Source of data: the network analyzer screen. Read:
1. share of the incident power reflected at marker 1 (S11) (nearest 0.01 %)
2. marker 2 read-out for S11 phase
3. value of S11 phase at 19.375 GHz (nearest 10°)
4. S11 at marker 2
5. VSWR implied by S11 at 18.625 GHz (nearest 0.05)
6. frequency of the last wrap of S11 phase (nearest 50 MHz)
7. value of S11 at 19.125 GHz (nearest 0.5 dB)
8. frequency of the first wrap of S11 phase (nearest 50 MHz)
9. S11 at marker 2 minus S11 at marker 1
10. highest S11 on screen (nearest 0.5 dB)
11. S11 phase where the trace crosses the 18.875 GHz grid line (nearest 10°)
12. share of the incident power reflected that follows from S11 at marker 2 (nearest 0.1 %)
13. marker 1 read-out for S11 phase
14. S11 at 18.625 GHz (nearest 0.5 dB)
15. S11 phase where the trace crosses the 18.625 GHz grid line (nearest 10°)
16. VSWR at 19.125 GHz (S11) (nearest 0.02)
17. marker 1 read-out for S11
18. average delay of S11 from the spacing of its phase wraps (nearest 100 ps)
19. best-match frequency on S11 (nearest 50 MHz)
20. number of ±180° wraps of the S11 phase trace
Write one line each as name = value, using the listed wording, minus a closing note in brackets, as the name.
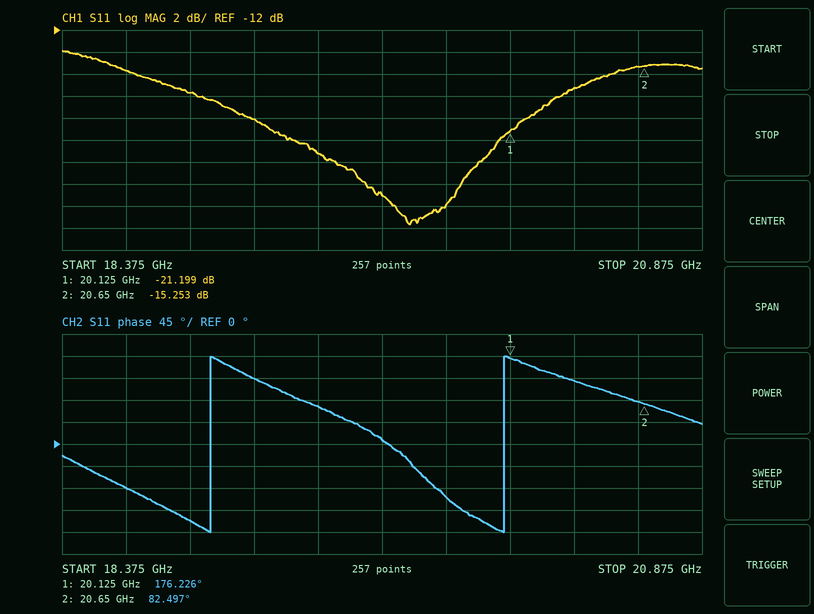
share of the incident power reflected at marker 1 (S11) = 0.76 %
marker 2 read-out for S11 phase = 82.497°
value of S11 phase at 19.375 GHz = 80°
S11 at marker 2 = -15.253 dB
VSWR implied by S11 at 18.625 GHz = 1.40
frequency of the last wrap of S11 phase = 20.10 GHz
value of S11 at 19.125 GHz = -20.0 dB
frequency of the first wrap of S11 phase = 18.95 GHz
S11 at marker 2 minus S11 at marker 1 = 5.946 dB
highest S11 on screen = -14.0 dB
S11 phase where the trace crosses the 18.875 GHz grid line = -160°
share of the incident power reflected that follows from S11 at marker 2 = 3.0 %
marker 1 read-out for S11 phase = 176.226°
S11 at 18.625 GHz = -15.5 dB
S11 phase where the trace crosses the 18.625 GHz grid line = -90°
VSWR at 19.125 GHz (S11) = 1.22
marker 1 read-out for S11 = -21.199 dB
average delay of S11 from the spacing of its phase wraps = 900 ps
best-match frequency on S11 = 19.75 GHz
number of ±180° wraps of the S11 phase trace = 2
